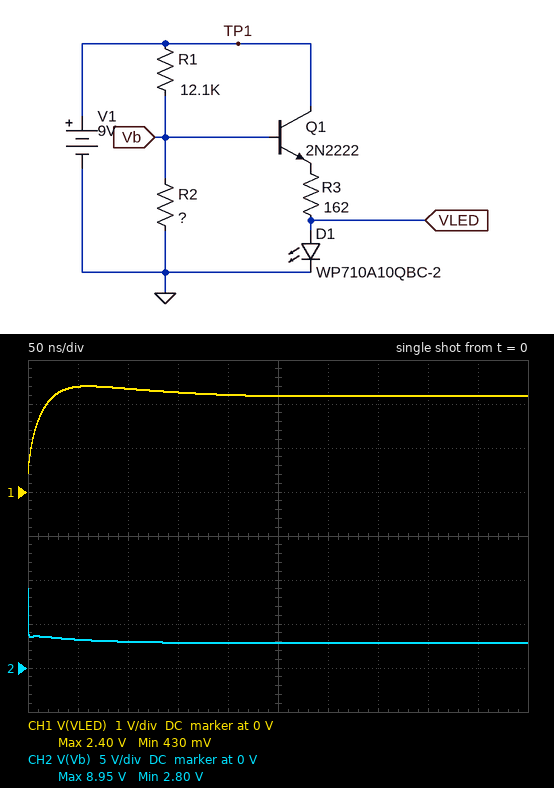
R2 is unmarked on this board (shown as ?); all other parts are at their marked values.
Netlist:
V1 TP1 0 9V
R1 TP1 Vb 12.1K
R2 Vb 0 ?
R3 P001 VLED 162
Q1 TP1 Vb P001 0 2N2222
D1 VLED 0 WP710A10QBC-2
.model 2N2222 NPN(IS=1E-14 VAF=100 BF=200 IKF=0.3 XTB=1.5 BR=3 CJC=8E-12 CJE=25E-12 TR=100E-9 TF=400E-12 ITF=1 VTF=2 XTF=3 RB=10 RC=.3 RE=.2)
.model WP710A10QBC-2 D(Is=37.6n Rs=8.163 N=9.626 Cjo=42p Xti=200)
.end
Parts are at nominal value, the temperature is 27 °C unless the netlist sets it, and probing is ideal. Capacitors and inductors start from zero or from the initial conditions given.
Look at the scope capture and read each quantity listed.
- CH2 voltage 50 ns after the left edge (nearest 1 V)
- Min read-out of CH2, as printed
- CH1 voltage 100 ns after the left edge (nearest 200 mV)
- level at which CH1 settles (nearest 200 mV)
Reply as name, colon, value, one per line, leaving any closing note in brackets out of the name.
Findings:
CH2 voltage 50 ns after the left edge: 3 V
Min read-out of CH2, as printed: 2.80 V
CH1 voltage 100 ns after the left edge: 2.4 V
level at which CH1 settles: 2.2 V
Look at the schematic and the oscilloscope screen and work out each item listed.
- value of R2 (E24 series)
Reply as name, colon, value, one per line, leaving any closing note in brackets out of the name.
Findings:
value of R2: 5.6 kΩ
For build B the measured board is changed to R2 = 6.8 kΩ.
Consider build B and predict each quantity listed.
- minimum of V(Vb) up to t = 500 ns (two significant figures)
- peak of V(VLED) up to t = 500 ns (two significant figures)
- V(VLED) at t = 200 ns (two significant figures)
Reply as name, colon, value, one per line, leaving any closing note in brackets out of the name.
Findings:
minimum of V(Vb) up to t = 500 ns: 3.2 V
peak of V(VLED) up to t = 500 ns: 2.6 V
V(VLED) at t = 200 ns: 2.5 V
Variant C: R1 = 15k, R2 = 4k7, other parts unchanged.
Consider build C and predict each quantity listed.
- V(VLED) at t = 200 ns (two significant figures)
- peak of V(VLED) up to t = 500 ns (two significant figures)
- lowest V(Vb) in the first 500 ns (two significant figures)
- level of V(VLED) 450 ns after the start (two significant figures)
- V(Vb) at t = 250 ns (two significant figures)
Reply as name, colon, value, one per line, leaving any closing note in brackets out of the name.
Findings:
V(VLED) at t = 200 ns: 1.9 V
peak of V(VLED) up to t = 500 ns: 2.0 V
lowest V(Vb) in the first 500 ns: 2.1 V
level of V(VLED) 450 ns after the start: 1.8 V
V(Vb) at t = 250 ns: 2.2 V
